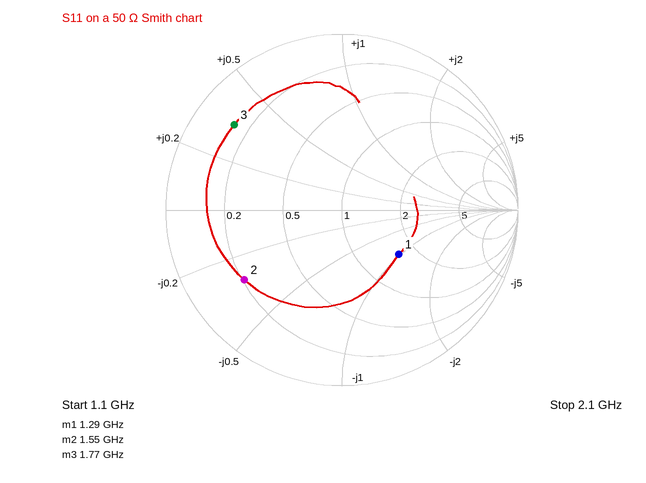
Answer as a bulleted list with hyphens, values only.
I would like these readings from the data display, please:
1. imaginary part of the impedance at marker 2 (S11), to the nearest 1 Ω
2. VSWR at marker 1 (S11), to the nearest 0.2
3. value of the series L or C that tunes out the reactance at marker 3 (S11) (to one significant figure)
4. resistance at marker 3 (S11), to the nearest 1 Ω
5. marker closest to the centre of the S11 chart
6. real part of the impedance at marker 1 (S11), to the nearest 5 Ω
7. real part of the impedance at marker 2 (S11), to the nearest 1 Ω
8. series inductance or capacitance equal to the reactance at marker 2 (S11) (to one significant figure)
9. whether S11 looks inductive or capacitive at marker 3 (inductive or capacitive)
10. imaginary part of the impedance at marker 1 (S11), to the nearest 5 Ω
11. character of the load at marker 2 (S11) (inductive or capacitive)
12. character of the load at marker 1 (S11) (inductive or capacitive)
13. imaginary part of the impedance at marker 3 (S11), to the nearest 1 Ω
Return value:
- -15 Ω
- 2.4
- 5 pF
- 7 Ω
- marker 1
- 80 Ω
- 10 Ω
- 7 pF
- inductive
- -50 Ω
- capacitive
- capacitive
- +17 Ω
